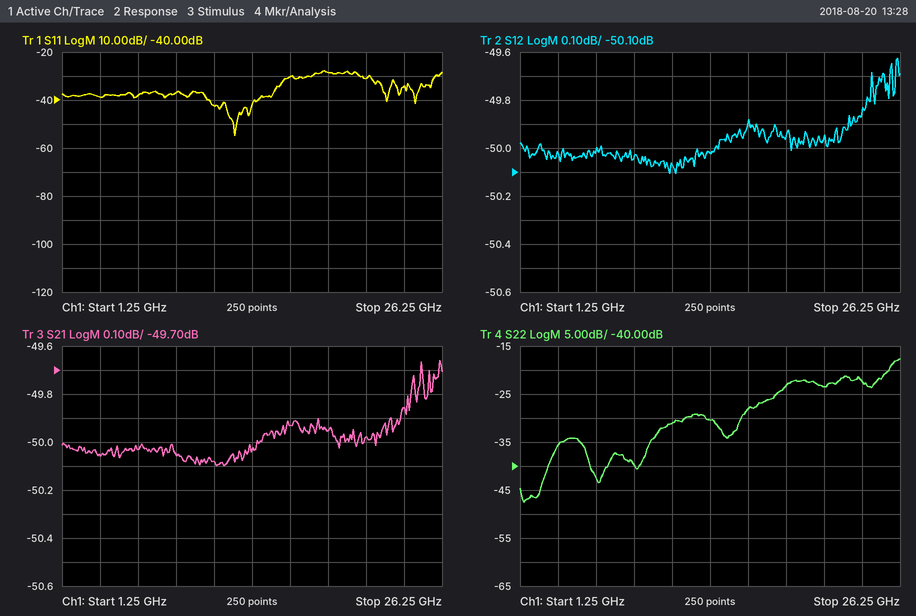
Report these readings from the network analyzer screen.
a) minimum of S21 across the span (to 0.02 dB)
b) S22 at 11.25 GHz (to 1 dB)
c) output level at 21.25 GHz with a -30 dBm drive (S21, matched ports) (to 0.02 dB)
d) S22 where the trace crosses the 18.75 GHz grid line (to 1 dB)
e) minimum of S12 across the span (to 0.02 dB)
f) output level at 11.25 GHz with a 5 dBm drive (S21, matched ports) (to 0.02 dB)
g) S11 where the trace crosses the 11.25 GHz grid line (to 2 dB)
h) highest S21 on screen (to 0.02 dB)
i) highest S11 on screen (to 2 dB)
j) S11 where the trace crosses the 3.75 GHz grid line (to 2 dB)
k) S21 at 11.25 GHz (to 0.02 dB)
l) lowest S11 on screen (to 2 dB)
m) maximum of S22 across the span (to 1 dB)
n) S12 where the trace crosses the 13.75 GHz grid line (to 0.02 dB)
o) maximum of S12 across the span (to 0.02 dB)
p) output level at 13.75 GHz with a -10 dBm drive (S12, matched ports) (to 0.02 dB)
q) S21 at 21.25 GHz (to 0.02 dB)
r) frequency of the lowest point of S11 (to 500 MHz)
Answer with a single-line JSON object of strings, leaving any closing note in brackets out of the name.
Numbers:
{"minimum of S21 across the span": "-50.10 dB", "S22 at 11.25 GHz": "-31 dB", "output level at 21.25 GHz with a -30 dBm drive (S21, matched ports)": "-79.98 dBm", "S22 where the trace crosses the 18.75 GHz grid line": "-23 dB", "minimum of S12 across the span": "-50.10 dB", "output level at 11.25 GHz with a 5 dBm drive (S21, matched ports)": "-45.08 dBm", "S11 where the trace crosses the 11.25 GHz grid line": "-42 dB", "highest S21 on screen": "-49.66 dB", "highest S11 on screen": "-28 dB", "S11 where the trace crosses the 3.75 GHz grid line": "-38 dB", "S21 at 11.25 GHz": "-50.08 dB", "lowest S11 on screen": "-54 dB", "maximum of S22 across the span": "-18 dB", "S12 where the trace crosses the 13.75 GHz grid line": "-50.02 dB", "maximum of S12 across the span": "-49.62 dB", "output level at 13.75 GHz with a -10 dBm drive (S12, matched ports)": "-60.02 dBm", "S21 at 21.25 GHz": "-49.98 dB", "frequency of the lowest point of S11": "12.5 GHz"}
